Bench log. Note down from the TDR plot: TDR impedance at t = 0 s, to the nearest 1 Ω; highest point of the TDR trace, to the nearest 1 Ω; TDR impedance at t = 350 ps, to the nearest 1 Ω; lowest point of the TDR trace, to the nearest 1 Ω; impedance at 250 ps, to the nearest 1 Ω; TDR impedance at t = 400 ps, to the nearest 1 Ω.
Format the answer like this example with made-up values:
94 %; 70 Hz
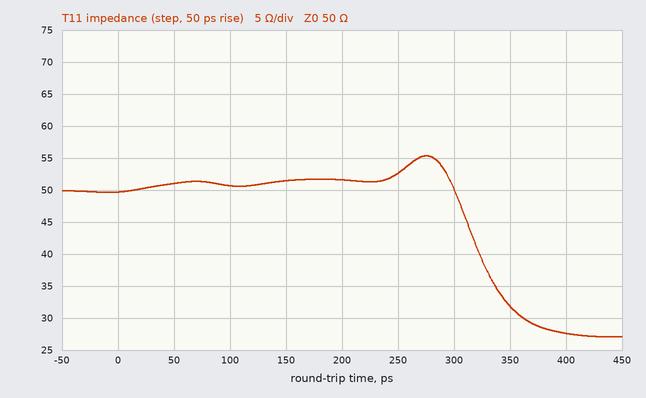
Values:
50 Ω; 55 Ω; 32 Ω; 27 Ω; 53 Ω; 28 Ω
